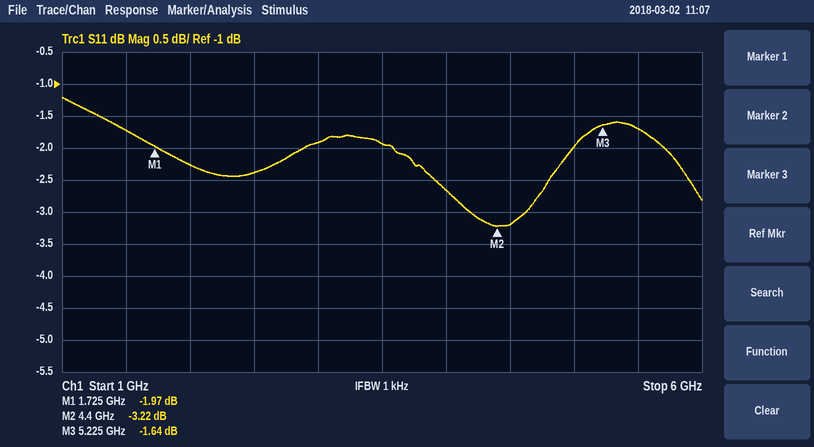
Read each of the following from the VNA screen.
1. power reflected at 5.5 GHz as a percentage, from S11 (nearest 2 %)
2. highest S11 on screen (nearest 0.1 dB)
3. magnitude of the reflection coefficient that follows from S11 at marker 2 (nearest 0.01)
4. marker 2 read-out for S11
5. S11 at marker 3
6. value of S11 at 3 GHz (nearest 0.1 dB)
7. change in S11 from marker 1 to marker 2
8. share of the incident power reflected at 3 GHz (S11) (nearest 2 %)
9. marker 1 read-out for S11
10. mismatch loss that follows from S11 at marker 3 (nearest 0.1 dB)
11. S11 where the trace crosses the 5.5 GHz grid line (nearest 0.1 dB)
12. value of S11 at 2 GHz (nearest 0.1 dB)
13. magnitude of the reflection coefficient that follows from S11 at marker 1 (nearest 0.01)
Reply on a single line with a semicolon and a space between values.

68 %; -1.2 dB; 0.69; -3.22 dB; -1.64 dB; -1.9 dB; -1.25 dB; 64 %; -1.97 dB; 5.0 dB; -1.7 dB; -2.3 dB; 0.80
